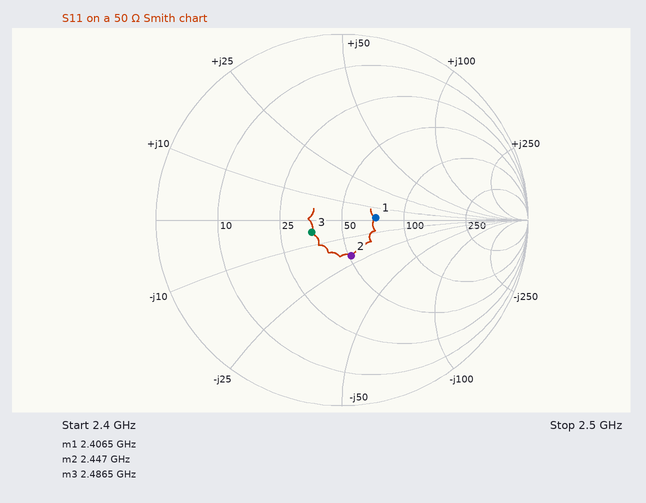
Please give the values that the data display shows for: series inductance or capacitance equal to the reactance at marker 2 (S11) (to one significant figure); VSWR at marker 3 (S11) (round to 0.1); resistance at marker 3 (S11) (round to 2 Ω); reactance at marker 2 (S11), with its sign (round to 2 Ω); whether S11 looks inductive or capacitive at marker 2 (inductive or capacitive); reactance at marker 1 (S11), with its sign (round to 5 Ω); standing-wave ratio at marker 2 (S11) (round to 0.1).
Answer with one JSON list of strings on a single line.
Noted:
["3 pF", "1.4", "36 Ω", "-20 Ω", "capacitive", "0 Ω", "1.5"]
